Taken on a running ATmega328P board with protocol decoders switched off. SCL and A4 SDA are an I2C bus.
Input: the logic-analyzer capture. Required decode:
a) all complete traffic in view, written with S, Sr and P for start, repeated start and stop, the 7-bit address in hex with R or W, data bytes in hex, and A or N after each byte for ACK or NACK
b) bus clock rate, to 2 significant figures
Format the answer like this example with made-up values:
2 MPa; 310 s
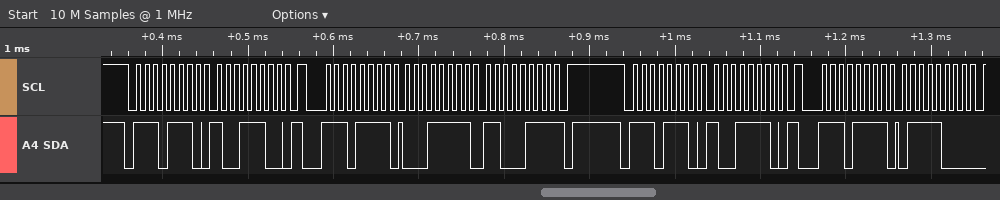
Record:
S 77W A 9C A Sr 77R A 1F A C7 N P S 77W A 9E A Sr 77R A 78 A; 100 kHz
